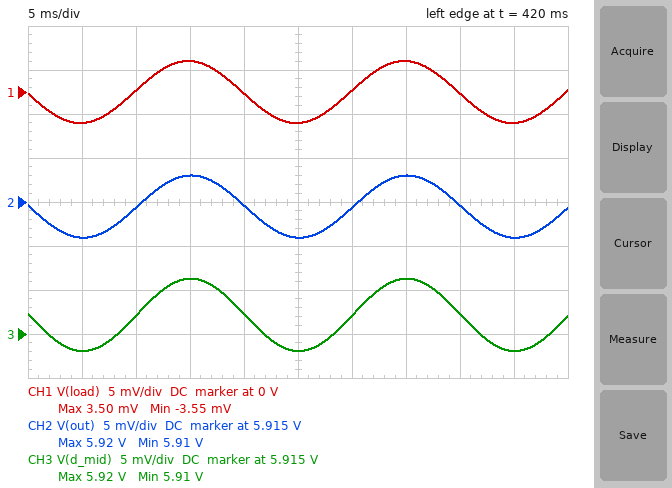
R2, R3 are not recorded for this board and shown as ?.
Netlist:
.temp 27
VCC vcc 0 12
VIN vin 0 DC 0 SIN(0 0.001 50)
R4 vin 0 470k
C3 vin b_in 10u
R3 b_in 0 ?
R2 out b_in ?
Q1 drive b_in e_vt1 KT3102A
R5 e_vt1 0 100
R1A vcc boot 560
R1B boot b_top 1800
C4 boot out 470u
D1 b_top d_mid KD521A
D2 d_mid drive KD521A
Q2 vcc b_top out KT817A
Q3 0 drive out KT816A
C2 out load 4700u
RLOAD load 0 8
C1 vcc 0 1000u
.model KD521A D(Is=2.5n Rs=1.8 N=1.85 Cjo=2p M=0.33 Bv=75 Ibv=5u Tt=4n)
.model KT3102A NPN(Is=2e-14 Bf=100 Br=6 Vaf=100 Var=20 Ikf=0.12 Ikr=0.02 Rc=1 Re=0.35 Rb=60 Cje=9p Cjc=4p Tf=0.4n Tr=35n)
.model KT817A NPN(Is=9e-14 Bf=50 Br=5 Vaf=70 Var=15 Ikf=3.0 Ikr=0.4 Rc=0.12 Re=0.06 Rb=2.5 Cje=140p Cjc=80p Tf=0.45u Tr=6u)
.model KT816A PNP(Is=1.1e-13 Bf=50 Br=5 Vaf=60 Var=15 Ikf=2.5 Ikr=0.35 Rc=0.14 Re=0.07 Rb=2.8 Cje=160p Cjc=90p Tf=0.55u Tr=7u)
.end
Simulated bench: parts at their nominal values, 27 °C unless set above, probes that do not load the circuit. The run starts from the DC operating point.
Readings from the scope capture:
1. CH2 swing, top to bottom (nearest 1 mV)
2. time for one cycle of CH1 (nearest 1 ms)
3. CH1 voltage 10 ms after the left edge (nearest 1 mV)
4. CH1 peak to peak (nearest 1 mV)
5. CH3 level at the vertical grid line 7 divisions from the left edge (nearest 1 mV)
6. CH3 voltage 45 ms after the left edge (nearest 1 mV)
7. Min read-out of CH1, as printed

7 mV
20 ms
0 V
7 mV
5.921 V
5.913 V
-3.55 mV
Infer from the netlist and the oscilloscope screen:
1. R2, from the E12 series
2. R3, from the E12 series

100 kΩ
33 kΩ
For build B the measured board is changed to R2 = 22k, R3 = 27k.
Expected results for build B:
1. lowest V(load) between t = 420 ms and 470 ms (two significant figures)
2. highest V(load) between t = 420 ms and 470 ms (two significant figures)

-3.6 mV
3.6 mV
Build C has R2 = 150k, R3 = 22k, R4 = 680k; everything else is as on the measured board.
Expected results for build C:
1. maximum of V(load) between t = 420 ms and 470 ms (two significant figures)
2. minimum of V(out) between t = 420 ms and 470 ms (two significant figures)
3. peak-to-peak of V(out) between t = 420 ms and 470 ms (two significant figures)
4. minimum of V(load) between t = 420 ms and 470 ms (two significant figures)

3.2 mV
8.1 V
6.4 mV
-3.2 mV
